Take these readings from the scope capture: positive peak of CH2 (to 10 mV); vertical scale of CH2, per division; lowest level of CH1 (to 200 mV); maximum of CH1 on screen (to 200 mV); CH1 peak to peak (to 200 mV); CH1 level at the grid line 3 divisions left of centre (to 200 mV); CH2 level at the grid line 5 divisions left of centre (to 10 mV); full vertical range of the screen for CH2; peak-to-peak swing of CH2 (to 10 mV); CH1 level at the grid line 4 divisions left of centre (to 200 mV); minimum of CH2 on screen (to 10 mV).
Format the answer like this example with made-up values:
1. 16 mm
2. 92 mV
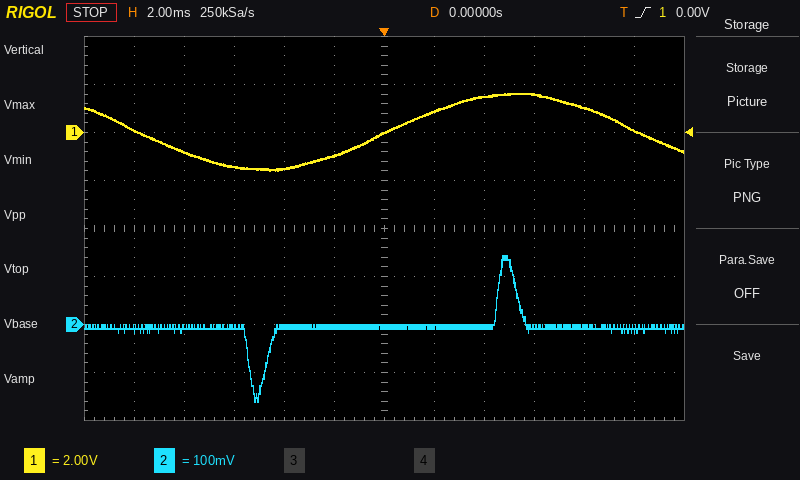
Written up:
1. 140 mV
2. 100 mV
3. -1.6 V
4. 1.6 V
5. 3.2 V
6. -1.4 V
7. -10 mV
8. 800 mV
9. 300 mV
10. -800 mV
11. -160 mV
